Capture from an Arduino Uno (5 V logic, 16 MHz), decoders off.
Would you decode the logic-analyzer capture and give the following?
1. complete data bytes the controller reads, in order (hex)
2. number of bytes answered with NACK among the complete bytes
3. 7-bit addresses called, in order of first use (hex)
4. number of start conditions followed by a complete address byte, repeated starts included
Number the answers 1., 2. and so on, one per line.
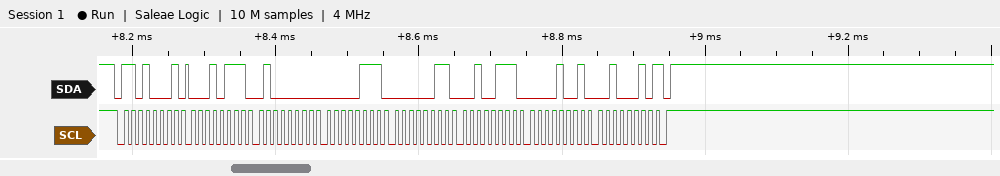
1. 17 40 07 03 27 09 22
2. 1
3. 0x68
4. 1
